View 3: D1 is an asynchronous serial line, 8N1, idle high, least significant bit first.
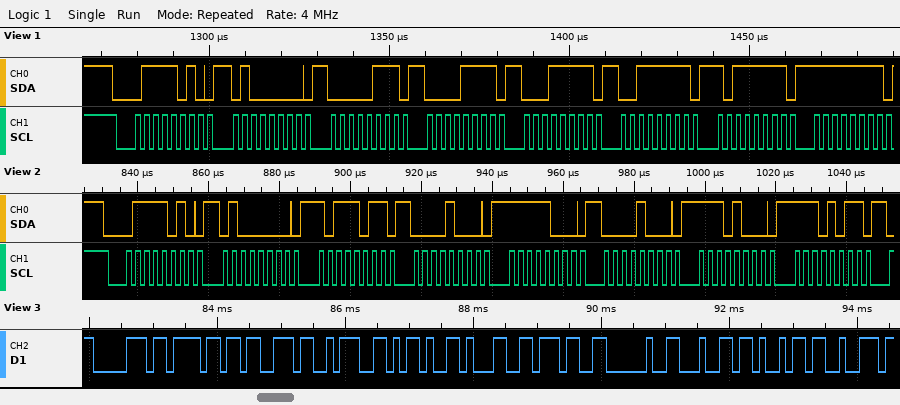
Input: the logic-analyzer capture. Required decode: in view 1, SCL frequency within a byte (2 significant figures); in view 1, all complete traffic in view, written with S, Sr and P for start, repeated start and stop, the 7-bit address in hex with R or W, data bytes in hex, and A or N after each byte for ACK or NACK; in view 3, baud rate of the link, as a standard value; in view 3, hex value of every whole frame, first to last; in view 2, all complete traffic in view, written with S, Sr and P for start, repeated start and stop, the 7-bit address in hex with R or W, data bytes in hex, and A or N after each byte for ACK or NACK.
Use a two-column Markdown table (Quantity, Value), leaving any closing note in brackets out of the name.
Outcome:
| Quantity | Value |
|---|---|
| in view 1, SCL frequency within a byte | 400 kHz |
| in view 1, all complete traffic in view, written with S, Sr and P for start, repeated start and stop, the 7-bit address in hex with R or W, data bytes in hex, and A or N after each byte for ACK or NACK | S 3DW A 40 A 07 A 0F A 1F A 3F A BF A FF A |
| in view 3, baud rate of the link, as a standard value | 9600 baud |
| in view 3, hex value of every whole frame, first to last | 70 6F 73 3A 2D 31 37 20 64 69 72 |
| in view 2, all complete traffic in view, written with S, Sr and P for start, repeated start and stop, the 7-bit address in hex with R or W, data bytes in hex, and A or N after each byte for ACK or NACK | S 3DW A 40 A BB A 08 A F8 A 08 A E8 A EB A |
